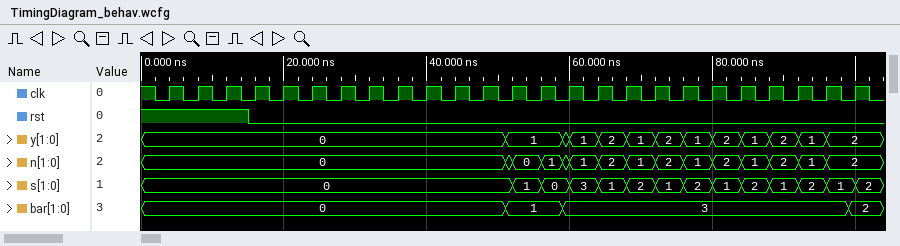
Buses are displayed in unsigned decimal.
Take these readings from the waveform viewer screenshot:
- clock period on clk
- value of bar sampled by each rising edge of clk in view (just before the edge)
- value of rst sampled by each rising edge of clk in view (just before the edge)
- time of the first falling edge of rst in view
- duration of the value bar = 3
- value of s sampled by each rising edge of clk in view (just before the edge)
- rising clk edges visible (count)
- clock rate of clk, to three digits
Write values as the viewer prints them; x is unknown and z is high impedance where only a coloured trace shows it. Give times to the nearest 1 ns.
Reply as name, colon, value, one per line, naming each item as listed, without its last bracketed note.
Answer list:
clock period on clk: 4 ns
value of bar sampled by each rising edge of clk in view: 0, 0, 0, 0, 0, 0, 0, 0, 0, 0, 0, 0, 1, 1, 3, 3, 3, 3, 3, 3, 3, 3, 3, 3, 2
value of rst sampled by each rising edge of clk in view: 1 1 1 0 0 0 0 0 0 0 0 0 0 0 0 0 0 0 0 0 0 0 0 0 0
time of the first falling edge of rst in view: 15 ns
duration of the value bar = 3: 40 ns
value of s sampled by each rising edge of clk in view: 0, 0, 0, 0, 0, 0, 0, 0, 0, 0, 0, 0, 0, 1, 0, 3, 1, 2, 1, 2, 1, 2, 1, 2, 1
rising clk edges visible: 25
clock rate of clk, to three digits: 250 MHz
